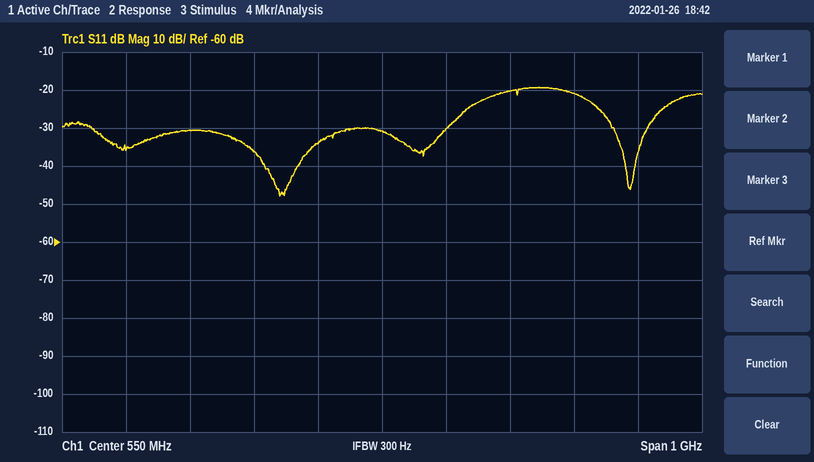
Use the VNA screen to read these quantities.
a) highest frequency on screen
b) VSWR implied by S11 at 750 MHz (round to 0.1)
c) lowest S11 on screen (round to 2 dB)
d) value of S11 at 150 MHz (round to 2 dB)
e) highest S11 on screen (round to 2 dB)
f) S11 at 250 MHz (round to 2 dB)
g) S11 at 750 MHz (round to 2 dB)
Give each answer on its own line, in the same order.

1.05 GHz
1.2
-48 dB
-36 dB
-20 dB
-30 dB
-20 dB
